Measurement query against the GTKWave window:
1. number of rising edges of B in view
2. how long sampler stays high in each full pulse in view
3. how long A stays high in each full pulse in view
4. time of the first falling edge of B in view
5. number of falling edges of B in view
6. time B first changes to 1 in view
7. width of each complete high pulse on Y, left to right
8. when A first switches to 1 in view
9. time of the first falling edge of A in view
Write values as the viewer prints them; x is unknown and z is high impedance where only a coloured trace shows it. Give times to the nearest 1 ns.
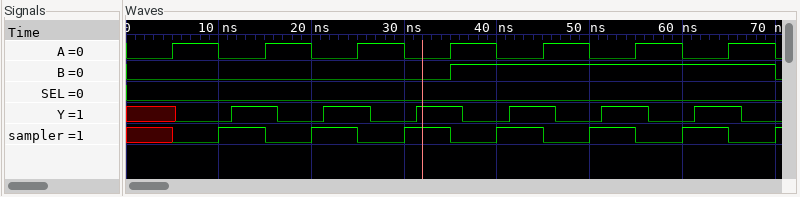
1
5 ns, 5 ns, 5 ns, 5 ns, 5 ns, 5 ns
5 ns, 5 ns, 5 ns, 5 ns, 5 ns, 5 ns, 5 ns
70 ns
1
35 ns
5 ns, 5 ns, 5 ns, 5 ns, 5 ns, 5 ns
5 ns
10 ns
